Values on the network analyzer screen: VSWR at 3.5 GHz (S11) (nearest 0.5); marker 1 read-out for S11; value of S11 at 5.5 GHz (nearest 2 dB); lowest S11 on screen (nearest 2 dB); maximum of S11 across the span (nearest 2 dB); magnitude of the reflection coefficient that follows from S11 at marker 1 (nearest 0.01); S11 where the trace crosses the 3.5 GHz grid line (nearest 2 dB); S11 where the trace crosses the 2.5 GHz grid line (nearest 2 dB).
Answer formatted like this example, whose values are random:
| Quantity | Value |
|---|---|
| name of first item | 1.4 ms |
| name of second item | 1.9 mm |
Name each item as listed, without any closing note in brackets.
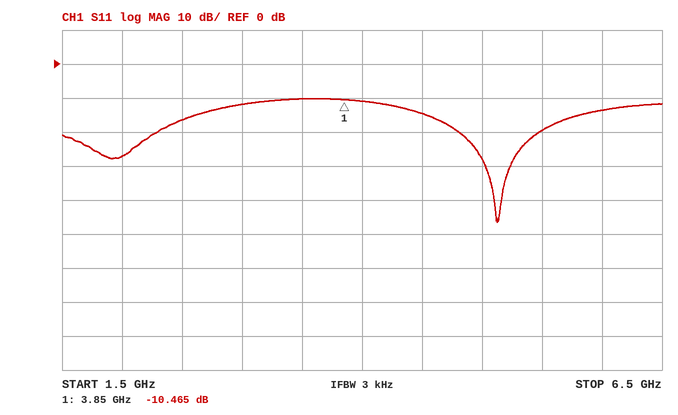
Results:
| Quantity | Value |
|---|---|
| VSWR at 3.5 GHz (S11) | 2.0 |
| marker 1 read-out for S11 | -10.465 dB |
| value of S11 at 5.5 GHz | -20 dB |
| lowest S11 on screen | -46 dB |
| maximum of S11 across the span | -10 dB |
| magnitude of the reflection coefficient that follows from S11 at marker 1 | 0.30 |
| S11 where the trace crosses the 3.5 GHz grid line | -10 dB |
| S11 where the trace crosses the 2.5 GHz grid line | -16 dB |
